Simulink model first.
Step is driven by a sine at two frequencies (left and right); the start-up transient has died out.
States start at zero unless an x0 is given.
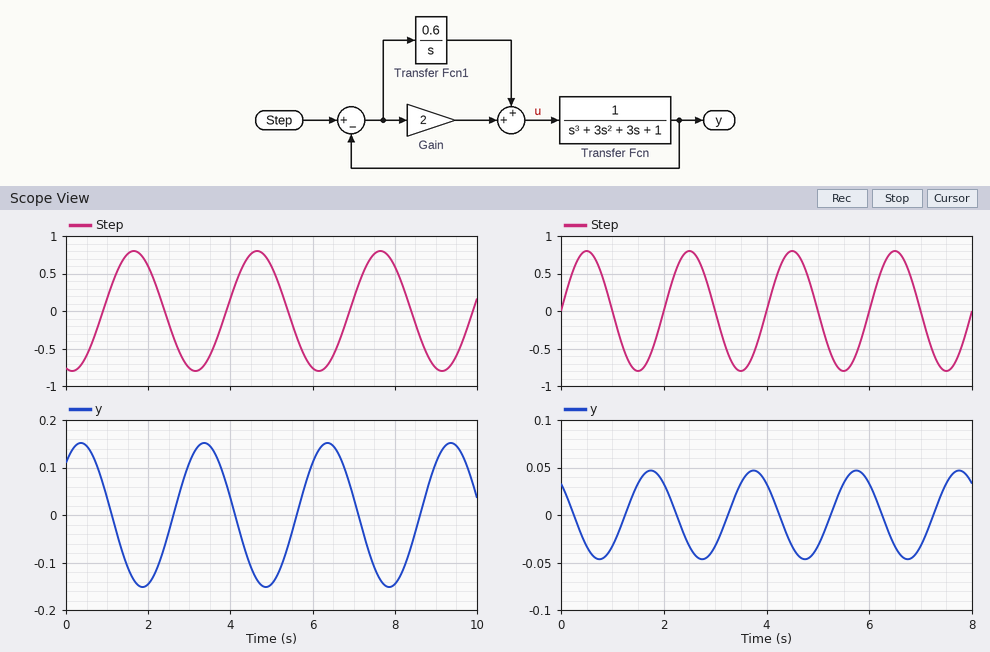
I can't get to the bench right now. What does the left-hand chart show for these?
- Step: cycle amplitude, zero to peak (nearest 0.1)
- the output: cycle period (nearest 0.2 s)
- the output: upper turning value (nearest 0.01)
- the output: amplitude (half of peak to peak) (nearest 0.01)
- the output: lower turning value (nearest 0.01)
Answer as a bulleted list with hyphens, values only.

- 0.8
- 3.0 s
- 0.15
- 0.15
- -0.15
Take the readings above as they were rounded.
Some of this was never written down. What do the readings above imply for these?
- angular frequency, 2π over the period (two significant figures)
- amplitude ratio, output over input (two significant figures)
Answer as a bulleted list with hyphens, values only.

- 2.1 rad/s
- 0.19
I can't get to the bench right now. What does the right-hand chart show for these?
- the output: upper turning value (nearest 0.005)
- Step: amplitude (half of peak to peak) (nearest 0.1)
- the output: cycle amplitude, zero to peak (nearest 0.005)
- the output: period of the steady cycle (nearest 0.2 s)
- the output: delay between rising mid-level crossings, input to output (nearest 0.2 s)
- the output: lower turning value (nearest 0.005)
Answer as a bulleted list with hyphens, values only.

- 0.045
- 0.8
- 0.045
- 2.0 s
- 1.2 s
- -0.045
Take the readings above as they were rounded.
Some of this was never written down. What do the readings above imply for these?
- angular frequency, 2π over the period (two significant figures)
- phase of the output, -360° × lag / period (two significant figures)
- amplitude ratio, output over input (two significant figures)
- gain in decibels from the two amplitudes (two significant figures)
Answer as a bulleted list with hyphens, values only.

- 3.1 rad/s
- -220°
- 0.056
- -25 dB
